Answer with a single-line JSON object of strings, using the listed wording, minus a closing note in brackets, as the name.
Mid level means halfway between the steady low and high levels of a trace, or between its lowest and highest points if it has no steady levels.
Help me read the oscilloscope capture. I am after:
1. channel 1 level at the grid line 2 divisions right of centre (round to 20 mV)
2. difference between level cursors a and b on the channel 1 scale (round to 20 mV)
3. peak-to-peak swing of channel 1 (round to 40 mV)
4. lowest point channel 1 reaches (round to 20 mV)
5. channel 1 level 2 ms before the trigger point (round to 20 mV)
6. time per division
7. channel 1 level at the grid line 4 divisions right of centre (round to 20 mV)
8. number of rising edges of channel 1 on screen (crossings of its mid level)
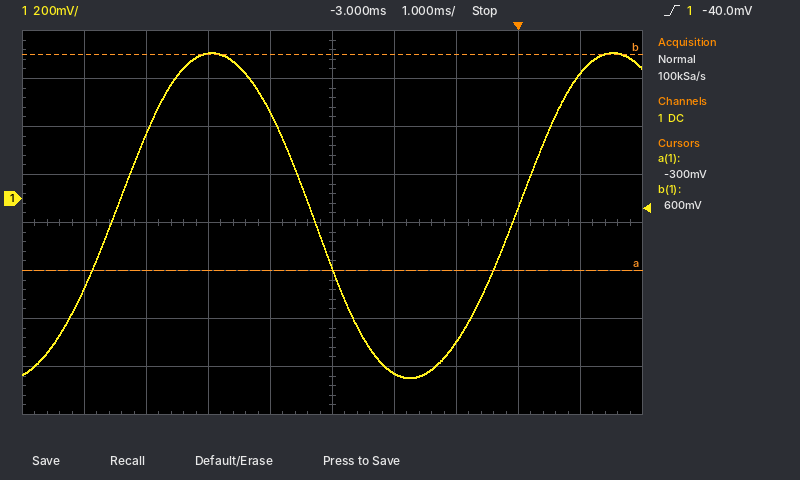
{"channel 1 level at the grid line 2 divisions right of centre": "-600 mV", "difference between level cursors a and b on the channel 1 scale": "900 mV", "peak-to-peak swing of channel 1": "1.36 V", "lowest point channel 1 reaches": "-740 mV", "channel 1 level 2 ms before the trigger point": "-720 mV", "time per division": "1 ms", "channel 1 level at the grid line 4 divisions right of centre": "520 mV", "number of rising edges of channel 1 on screen": "2"}
